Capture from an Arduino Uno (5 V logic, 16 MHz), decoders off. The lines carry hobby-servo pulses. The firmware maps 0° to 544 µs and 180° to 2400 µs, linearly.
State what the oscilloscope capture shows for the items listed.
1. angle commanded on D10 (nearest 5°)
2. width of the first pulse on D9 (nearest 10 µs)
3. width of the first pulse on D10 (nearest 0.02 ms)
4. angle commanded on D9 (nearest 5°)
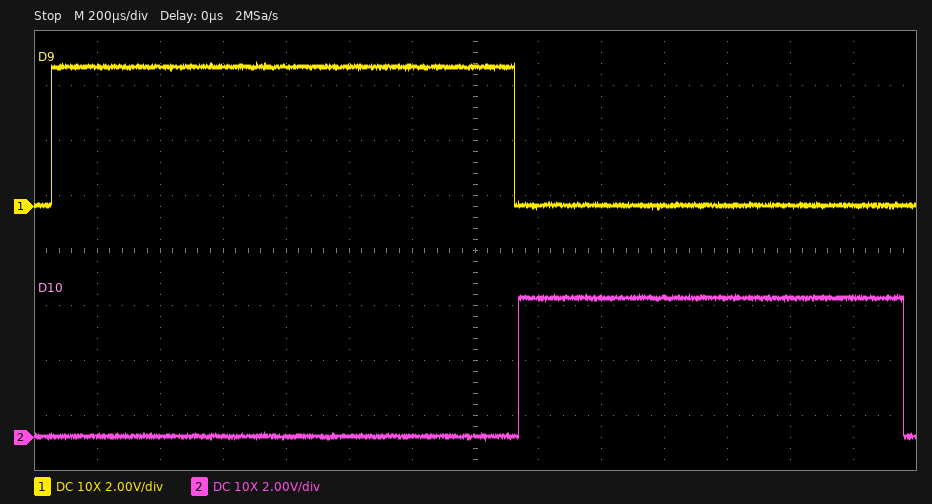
65°
1470 µs
1.22 ms
90°
